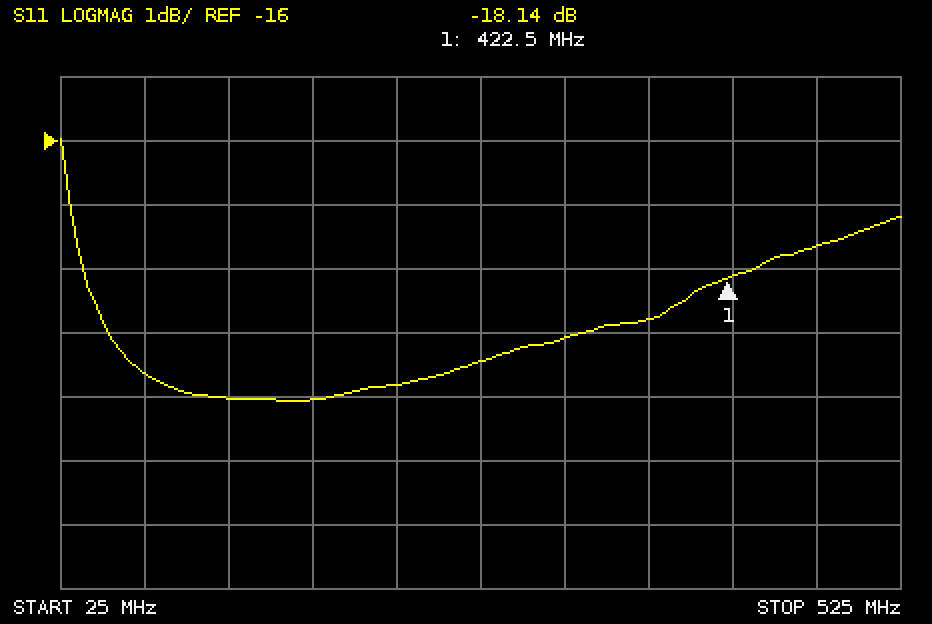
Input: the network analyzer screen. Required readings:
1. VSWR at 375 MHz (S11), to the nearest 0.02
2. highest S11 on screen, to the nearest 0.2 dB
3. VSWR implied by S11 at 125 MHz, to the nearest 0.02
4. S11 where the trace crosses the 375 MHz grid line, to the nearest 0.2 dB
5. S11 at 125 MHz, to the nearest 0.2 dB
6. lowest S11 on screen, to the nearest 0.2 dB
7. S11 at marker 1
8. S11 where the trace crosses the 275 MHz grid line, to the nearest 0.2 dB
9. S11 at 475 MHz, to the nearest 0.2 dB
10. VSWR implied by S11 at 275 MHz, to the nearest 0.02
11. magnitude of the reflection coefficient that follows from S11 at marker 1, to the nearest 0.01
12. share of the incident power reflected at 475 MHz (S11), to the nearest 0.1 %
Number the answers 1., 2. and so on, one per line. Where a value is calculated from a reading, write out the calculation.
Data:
1. |Γ| = 10^(-18.8/20) = 0.1148; VSWR = (1 + 0.1148)/(1 − 0.1148) ≈ 1.26
2. -16.0 dB
3. |Γ| = 10^(-20/20) = 0.1000; VSWR = (1 + 0.1000)/(1 − 0.1000) ≈ 1.22
4. -18.8 dB
5. -20.0 dB
6. -20.0 dB
7. -18.14 dB
8. -19.4 dB
9. -17.6 dB
10. |Γ| = 10^(-19.4/20) = 0.1072; VSWR = (1 + 0.1072)/(1 − 0.1072) ≈ 1.24
11. 10^(-18.14/20) ≈ 0.12
12. 10^(-17.6/10) ≈ 1.7 %
